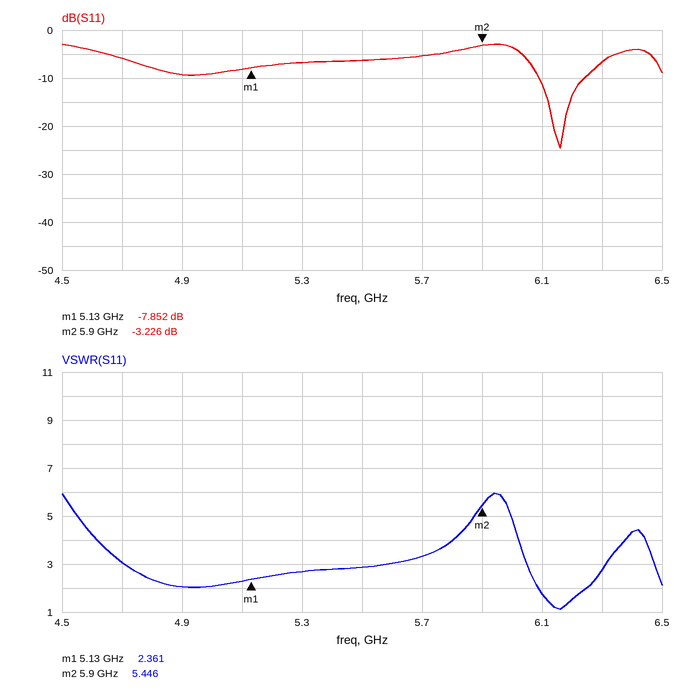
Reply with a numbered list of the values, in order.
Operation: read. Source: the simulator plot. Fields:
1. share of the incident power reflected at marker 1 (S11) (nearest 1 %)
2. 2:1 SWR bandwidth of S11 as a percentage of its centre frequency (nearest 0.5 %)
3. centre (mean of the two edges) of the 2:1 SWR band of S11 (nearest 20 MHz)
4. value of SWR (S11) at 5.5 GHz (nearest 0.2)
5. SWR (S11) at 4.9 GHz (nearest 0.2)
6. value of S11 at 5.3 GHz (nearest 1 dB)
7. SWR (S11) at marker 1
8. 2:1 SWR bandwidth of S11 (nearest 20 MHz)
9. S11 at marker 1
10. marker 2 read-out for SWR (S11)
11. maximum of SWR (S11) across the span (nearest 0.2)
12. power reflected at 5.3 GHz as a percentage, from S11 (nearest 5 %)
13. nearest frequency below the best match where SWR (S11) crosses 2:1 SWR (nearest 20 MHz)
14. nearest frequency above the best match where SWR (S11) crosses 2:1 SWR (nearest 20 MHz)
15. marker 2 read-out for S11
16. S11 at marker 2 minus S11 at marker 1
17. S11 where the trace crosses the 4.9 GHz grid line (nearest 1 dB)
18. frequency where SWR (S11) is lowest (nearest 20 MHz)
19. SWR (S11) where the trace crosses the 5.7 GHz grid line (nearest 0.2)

1. 16 %
2. 2.5 %
3. 6.16 GHz
4. 2.8
5. 2.0
6. -7 dB
7. 2.361
8. 160 MHz
9. -7.852 dB
10. 5.446
11. 6.0
12. 20 %
13. 6.08 GHz
14. 6.24 GHz
15. -3.226 dB
16. 4.626 dB
17. -9 dB
18. 6.16 GHz
19. 3.4
